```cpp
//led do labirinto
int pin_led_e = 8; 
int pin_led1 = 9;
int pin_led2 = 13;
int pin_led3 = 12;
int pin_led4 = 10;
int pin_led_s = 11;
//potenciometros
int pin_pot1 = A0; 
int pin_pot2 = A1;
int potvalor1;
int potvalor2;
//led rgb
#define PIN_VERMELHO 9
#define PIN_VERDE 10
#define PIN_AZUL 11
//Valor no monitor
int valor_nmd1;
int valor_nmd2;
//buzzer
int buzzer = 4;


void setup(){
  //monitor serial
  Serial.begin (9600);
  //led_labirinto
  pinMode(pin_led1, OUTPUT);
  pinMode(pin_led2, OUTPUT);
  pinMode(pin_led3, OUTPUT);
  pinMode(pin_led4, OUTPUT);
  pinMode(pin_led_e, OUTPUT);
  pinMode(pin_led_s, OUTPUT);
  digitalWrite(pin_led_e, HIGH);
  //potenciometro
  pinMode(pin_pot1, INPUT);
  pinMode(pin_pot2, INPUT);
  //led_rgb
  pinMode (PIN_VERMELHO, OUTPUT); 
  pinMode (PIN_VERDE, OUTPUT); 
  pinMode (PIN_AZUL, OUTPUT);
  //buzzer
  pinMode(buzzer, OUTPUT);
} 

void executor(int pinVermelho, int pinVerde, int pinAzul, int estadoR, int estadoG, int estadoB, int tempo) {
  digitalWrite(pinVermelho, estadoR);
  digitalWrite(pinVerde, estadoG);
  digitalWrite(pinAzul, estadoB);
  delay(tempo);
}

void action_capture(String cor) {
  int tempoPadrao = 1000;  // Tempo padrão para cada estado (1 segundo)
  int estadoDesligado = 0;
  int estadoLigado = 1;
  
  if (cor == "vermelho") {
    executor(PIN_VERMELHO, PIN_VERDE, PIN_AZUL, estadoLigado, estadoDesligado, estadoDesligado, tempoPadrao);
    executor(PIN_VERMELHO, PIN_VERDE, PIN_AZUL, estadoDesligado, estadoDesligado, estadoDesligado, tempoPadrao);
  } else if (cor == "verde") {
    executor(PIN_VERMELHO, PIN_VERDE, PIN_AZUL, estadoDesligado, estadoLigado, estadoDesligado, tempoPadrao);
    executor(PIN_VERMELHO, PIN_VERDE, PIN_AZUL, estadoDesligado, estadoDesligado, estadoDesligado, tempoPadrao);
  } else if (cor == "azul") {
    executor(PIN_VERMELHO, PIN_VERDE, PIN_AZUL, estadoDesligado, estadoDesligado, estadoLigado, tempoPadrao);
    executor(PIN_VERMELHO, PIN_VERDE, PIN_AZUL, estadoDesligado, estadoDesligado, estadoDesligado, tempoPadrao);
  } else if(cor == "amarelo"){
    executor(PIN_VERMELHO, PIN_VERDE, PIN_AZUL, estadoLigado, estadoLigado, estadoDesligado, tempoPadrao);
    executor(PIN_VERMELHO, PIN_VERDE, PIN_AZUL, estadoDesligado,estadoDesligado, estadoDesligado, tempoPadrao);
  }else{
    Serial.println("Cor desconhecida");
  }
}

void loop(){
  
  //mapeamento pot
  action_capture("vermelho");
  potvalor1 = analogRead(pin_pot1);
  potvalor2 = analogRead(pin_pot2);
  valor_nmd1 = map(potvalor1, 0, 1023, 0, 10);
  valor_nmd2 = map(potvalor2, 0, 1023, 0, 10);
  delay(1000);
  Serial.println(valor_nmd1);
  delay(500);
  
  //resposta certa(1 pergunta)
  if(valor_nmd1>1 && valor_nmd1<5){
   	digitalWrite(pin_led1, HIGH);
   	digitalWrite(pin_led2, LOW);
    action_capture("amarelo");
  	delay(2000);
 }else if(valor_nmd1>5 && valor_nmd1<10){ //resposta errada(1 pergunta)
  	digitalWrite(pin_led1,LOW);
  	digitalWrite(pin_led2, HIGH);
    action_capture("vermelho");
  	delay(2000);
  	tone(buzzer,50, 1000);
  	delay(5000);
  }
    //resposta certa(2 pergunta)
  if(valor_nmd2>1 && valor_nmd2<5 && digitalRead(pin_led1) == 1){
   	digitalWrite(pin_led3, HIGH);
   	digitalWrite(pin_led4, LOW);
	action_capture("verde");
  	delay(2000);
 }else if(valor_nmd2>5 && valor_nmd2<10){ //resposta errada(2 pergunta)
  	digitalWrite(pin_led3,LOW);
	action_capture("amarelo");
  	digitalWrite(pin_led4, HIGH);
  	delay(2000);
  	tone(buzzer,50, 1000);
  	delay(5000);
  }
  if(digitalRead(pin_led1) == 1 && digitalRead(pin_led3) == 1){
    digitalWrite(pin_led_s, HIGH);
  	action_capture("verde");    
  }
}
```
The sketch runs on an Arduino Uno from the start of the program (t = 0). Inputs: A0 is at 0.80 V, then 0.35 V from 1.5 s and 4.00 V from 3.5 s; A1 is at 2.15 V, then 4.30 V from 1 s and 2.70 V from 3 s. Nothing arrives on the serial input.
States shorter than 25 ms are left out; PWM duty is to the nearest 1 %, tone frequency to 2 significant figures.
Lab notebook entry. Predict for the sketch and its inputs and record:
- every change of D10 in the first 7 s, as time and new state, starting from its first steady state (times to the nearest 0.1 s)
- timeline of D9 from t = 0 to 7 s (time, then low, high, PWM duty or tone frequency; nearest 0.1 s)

0 s low; 3.5 s high; 4.5 s low; 5.5 s high
0 s high; 1 s low; 3.5 s high; 4.5 s low
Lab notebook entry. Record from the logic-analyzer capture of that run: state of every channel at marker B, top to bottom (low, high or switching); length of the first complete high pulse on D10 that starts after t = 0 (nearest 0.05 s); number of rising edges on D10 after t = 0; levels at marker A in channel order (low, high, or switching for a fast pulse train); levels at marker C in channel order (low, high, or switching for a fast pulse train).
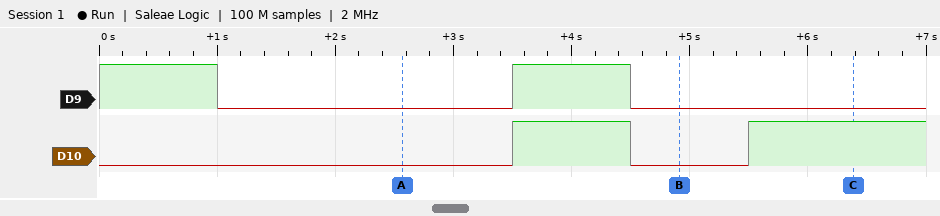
D9 low, D10 low
1.00 s
2
D9 low, D10 low
D9 low, D10 high
